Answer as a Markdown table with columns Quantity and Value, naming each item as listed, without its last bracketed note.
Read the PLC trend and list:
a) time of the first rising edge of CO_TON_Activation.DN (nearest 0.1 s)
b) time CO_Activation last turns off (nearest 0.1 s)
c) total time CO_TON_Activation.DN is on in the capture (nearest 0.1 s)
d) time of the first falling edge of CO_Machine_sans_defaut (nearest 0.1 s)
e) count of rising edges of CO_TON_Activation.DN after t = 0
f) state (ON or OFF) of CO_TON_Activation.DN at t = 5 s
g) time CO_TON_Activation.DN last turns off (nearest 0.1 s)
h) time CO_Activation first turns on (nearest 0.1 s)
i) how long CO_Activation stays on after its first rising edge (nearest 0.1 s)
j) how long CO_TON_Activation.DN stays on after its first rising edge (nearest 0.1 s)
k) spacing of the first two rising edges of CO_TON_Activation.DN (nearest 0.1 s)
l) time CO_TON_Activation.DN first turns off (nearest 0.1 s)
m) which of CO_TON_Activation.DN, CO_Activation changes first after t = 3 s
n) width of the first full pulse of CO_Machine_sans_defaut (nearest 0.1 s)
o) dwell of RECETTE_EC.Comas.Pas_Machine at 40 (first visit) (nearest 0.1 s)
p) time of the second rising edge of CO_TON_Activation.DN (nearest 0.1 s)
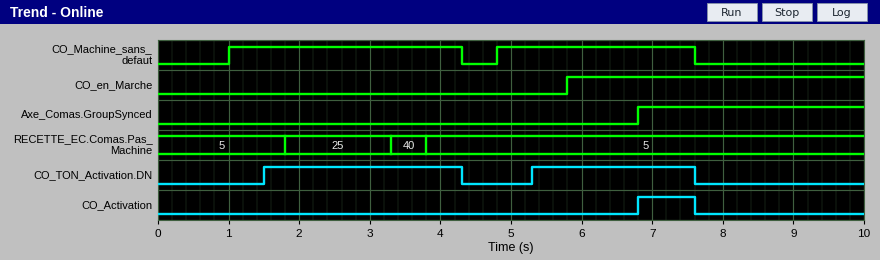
| Quantity | Value |
|---|---|
| time of the first rising edge of CO_TON_Activation.DN | 1.5 s |
| time CO_Activation last turns off | 7.6 s |
| total time CO_TON_Activation.DN is on in the capture | 5.1 s |
| time of the first falling edge of CO_Machine_sans_defaut | 4.3 s |
| count of rising edges of CO_TON_Activation.DN after t = 0 | 2 |
| state (ON or OFF) of CO_TON_Activation.DN at t = 5 s | OFF |
| time CO_TON_Activation.DN last turns off | 7.6 s |
| time CO_Activation first turns on | 6.8 s |
| how long CO_Activation stays on after its first rising edge | 0.8 s |
| how long CO_TON_Activation.DN stays on after its first rising edge | 2.8 s |
| spacing of the first two rising edges of CO_TON_Activation.DN | 3.8 s |
| time CO_TON_Activation.DN first turns off | 4.3 s |
| which of CO_TON_Activation.DN, CO_Activation changes first after t = 3 s | CO_TON_Activation.DN |
| width of the first full pulse of CO_Machine_sans_defaut | 3.3 s |
| dwell of RECETTE_EC.Comas.Pas_Machine at 40 (first visit) | 0.5 s |
| time of the second rising edge of CO_TON_Activation.DN | 5.3 s |
